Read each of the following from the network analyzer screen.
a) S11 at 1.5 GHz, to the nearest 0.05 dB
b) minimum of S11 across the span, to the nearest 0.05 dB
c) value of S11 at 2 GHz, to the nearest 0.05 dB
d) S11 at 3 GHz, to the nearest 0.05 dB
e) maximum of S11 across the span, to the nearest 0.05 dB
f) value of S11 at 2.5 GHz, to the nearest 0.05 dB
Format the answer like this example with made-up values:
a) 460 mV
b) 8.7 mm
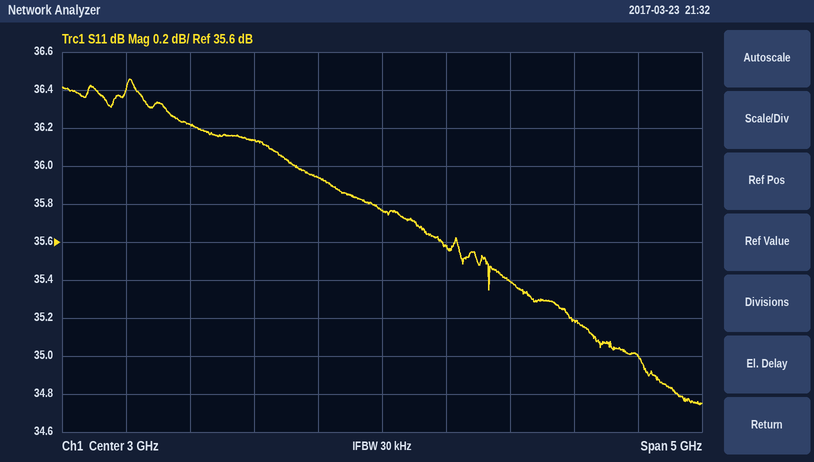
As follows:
a) 36.20 dB
b) 34.75 dB
c) 36.15 dB
d) 35.75 dB
e) 36.45 dB
f) 35.95 dB
